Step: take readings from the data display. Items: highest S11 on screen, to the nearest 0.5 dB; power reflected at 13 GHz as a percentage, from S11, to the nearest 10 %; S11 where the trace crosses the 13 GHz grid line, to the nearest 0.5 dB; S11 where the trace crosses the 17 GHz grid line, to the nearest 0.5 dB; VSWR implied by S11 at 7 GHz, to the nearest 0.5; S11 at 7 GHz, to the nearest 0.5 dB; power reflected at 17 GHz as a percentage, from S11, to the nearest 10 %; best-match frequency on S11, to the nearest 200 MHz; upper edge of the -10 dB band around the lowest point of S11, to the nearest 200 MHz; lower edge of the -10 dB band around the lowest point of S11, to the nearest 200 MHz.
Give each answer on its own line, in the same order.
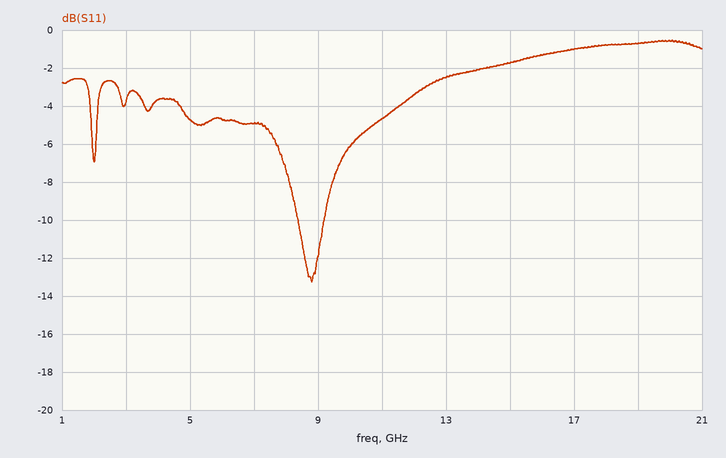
-0.5 dB
60 %
-2.5 dB
-1.0 dB
3.5
-5.0 dB
80 %
8.8 GHz
9.2 GHz
8.4 GHz
